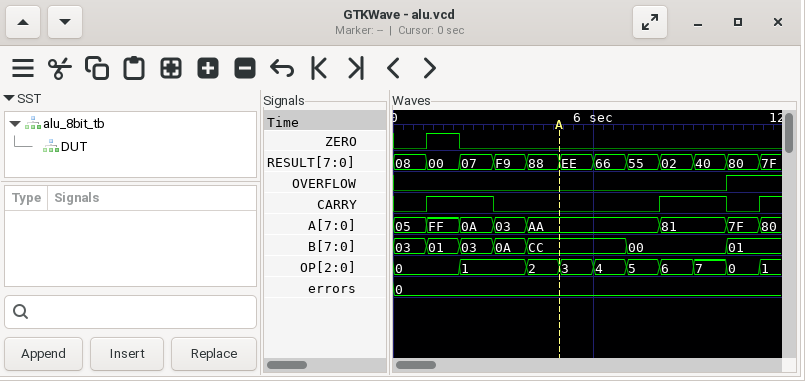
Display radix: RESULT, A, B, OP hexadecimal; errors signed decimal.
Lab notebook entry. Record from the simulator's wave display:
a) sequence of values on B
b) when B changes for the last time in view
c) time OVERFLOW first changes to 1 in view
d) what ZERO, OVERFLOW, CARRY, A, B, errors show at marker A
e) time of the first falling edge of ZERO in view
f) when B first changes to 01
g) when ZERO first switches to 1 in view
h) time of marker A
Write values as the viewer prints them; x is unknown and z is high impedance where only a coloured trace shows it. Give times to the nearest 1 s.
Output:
03, 01, 03, 0A, CC, 00, 01
10 s
10 s
ZERO=0, OVERFLOW=0, CARRY=0, A=AA, B=CC, errors=0
2 s
1 s
1 s
5 s
